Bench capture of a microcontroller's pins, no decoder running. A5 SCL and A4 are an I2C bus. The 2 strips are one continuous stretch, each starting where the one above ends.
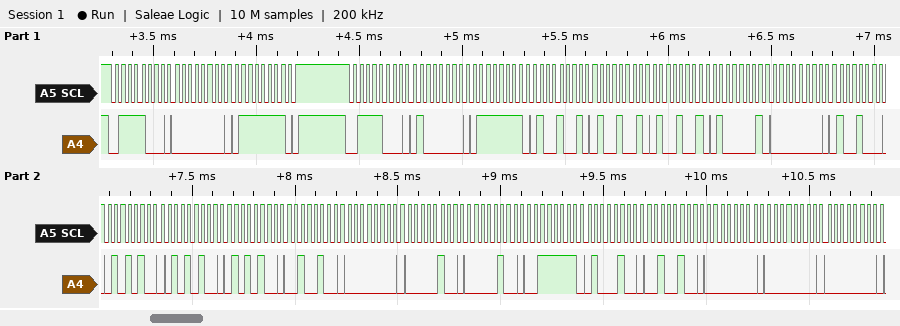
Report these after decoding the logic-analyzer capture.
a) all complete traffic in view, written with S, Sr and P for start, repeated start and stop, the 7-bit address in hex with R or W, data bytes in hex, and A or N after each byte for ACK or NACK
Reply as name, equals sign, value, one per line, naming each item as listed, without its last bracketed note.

all complete traffic in view, written with S, Sr and P for start, repeated start and stop, the 7-bit address in hex with R or W, data bytes in hex, and A or N after each byte for ACK or NACK = S 3CW A 00 A 7F A P S 3CW A 40 A 7F A 49 A 49 A 49 A 41 A 00 A 48 A 54 A 54 A 54 A 24 A 00 A 04 A 04 A 3F A 44 A 24 A 00 A 00 A 00 A
